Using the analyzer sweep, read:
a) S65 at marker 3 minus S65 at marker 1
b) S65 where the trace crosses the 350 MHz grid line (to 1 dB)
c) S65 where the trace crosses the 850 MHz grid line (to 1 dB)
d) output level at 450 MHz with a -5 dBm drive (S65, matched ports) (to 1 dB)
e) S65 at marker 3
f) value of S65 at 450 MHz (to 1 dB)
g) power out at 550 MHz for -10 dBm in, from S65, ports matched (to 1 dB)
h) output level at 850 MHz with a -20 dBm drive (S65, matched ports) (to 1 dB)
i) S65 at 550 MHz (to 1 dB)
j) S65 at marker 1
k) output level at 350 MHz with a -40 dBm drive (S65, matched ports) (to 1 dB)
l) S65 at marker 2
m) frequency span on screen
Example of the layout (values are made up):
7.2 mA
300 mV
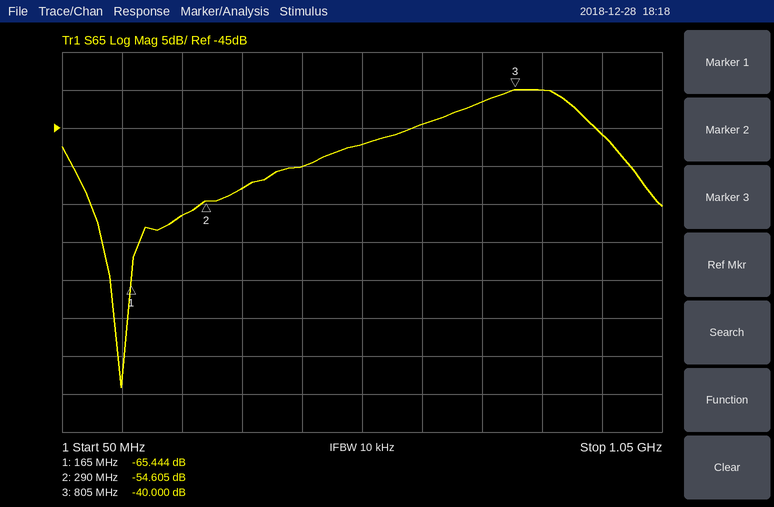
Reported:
25.444 dB
-53 dB
-40 dB
-55 dBm
-40.000 dB
-50 dB
-57 dBm
-60 dBm
-47 dB
-65.444 dB
-93 dBm
-54.605 dB
1 GHz
